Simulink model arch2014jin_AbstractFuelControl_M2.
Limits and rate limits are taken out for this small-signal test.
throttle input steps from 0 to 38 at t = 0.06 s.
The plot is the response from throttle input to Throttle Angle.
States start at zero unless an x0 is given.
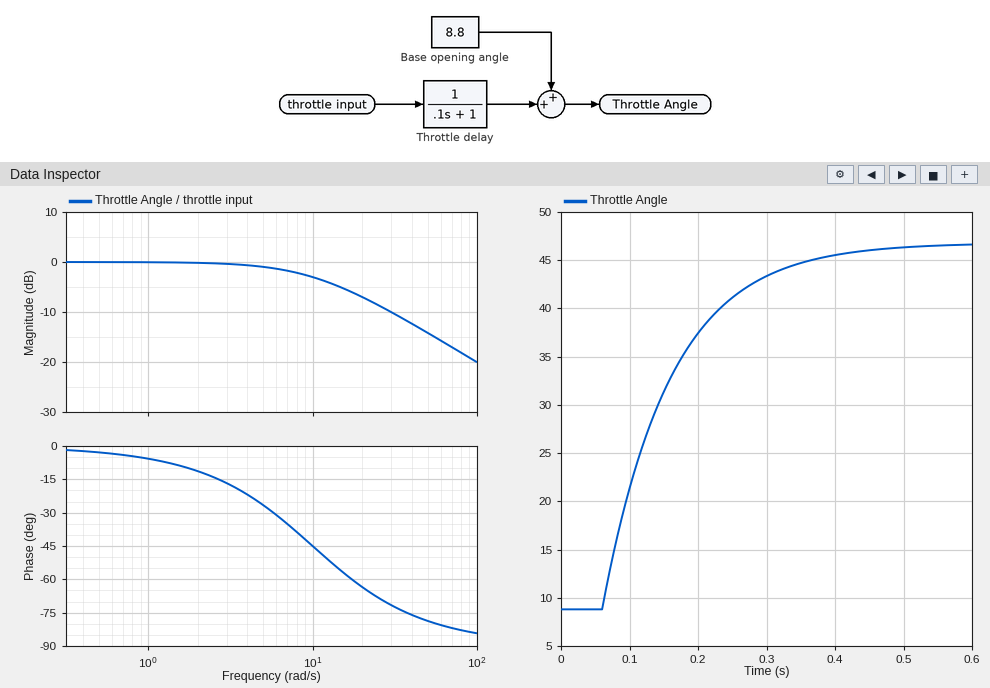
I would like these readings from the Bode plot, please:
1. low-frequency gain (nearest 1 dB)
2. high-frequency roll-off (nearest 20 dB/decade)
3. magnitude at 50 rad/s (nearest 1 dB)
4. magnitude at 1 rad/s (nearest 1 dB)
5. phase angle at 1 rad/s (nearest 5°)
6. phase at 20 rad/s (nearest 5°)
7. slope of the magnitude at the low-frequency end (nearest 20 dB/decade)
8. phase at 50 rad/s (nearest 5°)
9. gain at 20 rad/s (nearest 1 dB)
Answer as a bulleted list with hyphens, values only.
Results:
- 0 dB
- -20 dB/decade
- -14 dB
- 0 dB
- -5°
- -65°
- 0 dB/decade
- -80°
- -7 dB
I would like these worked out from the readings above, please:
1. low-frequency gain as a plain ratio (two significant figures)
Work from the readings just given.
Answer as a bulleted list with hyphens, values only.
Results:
- 1.0
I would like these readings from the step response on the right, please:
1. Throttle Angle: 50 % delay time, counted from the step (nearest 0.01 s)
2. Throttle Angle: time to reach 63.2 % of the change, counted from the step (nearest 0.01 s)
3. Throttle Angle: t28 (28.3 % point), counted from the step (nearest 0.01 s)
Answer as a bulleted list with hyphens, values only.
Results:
- 0.07 s
- 0.10 s
- 0.03 s
